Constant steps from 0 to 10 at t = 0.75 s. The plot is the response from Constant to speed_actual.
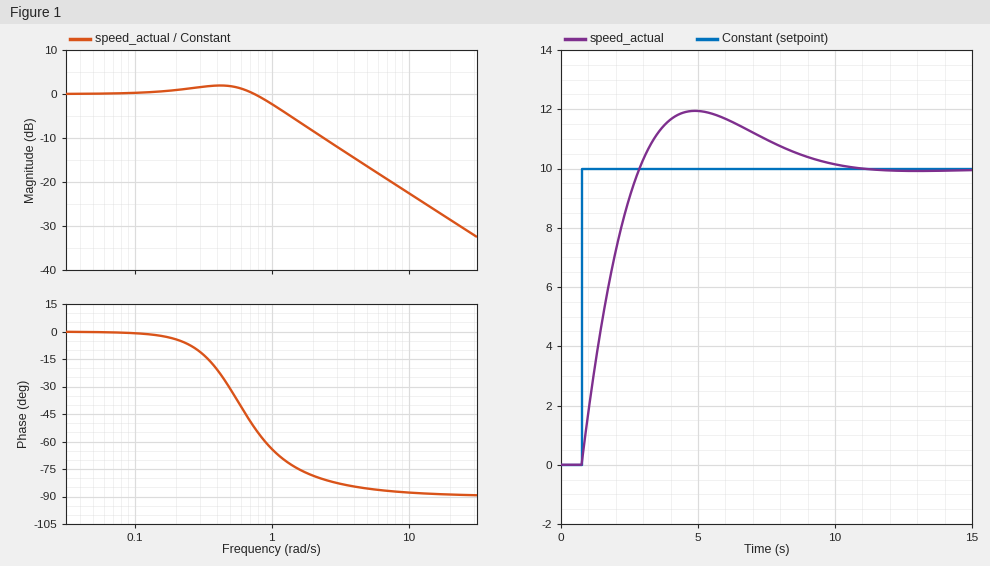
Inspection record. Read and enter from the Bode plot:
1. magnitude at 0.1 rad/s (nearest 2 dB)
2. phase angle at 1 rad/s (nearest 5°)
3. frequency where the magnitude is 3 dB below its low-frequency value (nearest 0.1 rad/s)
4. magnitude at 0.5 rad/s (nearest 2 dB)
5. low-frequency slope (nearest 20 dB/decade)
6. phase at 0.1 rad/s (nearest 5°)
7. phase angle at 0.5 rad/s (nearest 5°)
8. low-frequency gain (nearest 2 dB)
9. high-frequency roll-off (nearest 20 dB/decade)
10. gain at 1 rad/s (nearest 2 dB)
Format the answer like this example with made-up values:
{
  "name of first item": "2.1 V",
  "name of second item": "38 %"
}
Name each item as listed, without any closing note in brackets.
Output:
{
  "magnitude at 0.1 rad/s": "0 dB",
  "phase angle at 1 rad/s": "-65°",
  "frequency where the magnitude is 3 dB below its low-frequency value": "1.1 rad/s",
  "magnitude at 0.5 rad/s": "2 dB",
  "low-frequency slope": "0 dB/decade",
  "phase at 0.1 rad/s": "0°",
  "phase angle at 0.5 rad/s": "-30°",
  "low-frequency gain": "0 dB",
  "high-frequency roll-off": "-20 dB/decade",
  "gain at 1 rad/s": "-2 dB"
}
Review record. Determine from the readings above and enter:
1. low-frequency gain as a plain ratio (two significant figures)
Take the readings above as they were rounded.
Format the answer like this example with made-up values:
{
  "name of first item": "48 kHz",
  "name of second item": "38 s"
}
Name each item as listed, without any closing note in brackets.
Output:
{
  "low-frequency gain as a plain ratio": "1.0"
}
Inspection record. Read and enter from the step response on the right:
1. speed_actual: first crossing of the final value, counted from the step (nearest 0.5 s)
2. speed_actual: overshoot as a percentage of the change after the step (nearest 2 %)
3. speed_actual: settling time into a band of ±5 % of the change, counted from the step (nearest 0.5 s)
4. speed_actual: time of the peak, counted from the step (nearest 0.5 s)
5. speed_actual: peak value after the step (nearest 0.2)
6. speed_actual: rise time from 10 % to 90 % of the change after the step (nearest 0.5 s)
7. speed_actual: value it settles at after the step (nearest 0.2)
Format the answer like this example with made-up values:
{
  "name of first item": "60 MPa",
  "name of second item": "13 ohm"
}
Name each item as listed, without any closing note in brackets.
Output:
{
  "speed_actual: first crossing of the final value, counted from the step": "2.0 s",
  "speed_actual: overshoot as a percentage of the change after the step": "20 %",
  "speed_actual: settling time into a band of ±5 % of the change, counted from the step": "8.0 s",
  "speed_actual: time of the peak, counted from the step": "4.0 s",
  "speed_actual: peak value after the step": "12.0",
  "speed_actual: rise time from 10 % to 90 % of the change after the step": "1.5 s",
  "speed_actual: value it settles at after the step": "10.0"
}
